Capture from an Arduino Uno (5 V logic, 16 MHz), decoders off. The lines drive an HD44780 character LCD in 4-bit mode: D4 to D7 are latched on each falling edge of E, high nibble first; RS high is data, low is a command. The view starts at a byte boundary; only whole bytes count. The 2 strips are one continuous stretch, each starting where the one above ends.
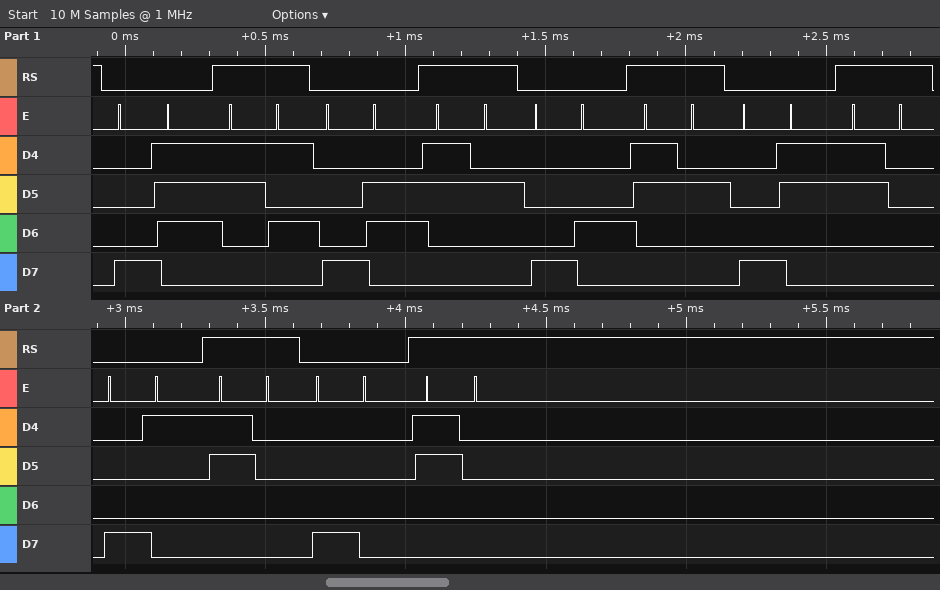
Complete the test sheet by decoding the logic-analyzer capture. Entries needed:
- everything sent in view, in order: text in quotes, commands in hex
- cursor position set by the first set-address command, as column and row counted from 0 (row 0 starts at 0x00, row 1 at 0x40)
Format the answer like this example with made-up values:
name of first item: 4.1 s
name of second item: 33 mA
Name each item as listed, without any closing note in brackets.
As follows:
everything sent in view, in order: text in quotes, commands in hex: 0x87 "5" 0x86 "2" 0x84 "2" 0x83 "0" 0x81 "0" 0x80 "0"
cursor position set by the first set-address command, as column and row counted from 0: column 7, row 0
